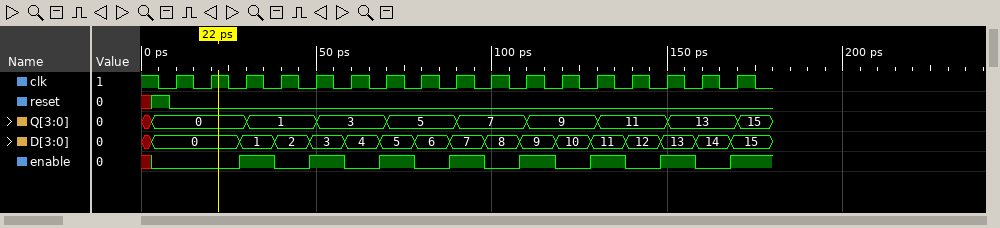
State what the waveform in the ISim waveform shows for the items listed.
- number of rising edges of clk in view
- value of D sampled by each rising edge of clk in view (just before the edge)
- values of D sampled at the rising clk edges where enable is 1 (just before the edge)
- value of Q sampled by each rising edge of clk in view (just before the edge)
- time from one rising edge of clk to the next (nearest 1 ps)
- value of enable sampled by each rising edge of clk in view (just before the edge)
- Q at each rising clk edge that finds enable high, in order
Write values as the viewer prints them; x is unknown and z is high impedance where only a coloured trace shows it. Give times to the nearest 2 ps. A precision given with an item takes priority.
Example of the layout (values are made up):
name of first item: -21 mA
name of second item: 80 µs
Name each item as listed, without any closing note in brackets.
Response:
number of rising edges of clk in view: 17
value of D sampled by each rising edge of clk in view: 0, 0, 1, 2, 3, 4, 5, 6, 7, 8, 9, 10, 11, 12, 13, 14, 15
values of D sampled at the rising clk edges where enable is 1: 1, 3, 5, 7, 9, 11, 13, 15
value of Q sampled by each rising edge of clk in view: 0, 0, 0, 1, 1, 3, 3, 5, 5, 7, 7, 9, 9, 11, 11, 13, 13
time from one rising edge of clk to the next: 10 ps
value of enable sampled by each rising edge of clk in view: 0 0 1 0 1 0 1 0 1 0 1 0 1 0 1 0 1
Q at each rising clk edge that finds enable high, in order: 0, 1, 3, 5, 7, 9, 11, 13
